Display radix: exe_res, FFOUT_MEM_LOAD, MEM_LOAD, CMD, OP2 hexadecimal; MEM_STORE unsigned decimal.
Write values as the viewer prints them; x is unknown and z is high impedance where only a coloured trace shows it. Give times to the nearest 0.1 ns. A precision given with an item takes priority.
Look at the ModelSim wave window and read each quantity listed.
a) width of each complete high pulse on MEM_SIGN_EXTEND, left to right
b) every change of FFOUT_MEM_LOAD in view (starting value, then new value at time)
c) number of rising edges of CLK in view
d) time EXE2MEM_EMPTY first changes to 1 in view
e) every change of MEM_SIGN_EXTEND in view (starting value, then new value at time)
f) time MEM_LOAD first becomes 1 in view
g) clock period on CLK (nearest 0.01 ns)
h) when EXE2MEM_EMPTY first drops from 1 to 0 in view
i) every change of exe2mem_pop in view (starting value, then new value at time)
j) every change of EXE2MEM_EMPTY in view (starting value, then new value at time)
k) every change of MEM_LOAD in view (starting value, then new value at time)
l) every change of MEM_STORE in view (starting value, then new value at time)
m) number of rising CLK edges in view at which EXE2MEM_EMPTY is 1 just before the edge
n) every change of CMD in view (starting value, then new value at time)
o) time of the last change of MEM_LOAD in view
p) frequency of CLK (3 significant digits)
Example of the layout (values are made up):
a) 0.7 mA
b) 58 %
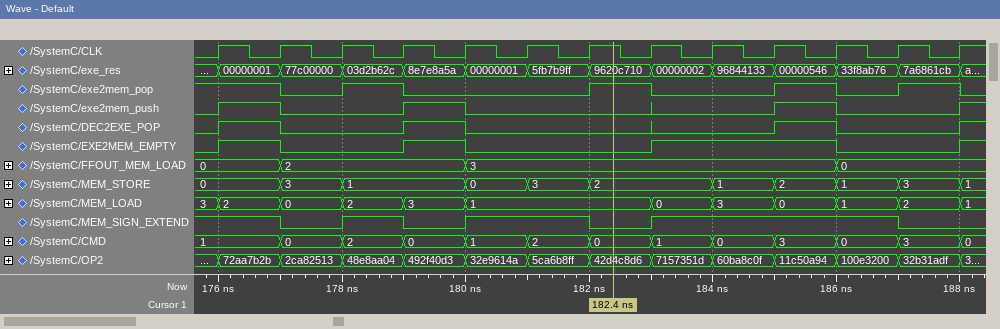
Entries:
a) 1 ns, 2 ns, 4 ns
b) 0, 2 at 177 ns, 3 at 180 ns, 0 at 186 ns
c) 13
d) 176 ns
e) 1, 0 at 177 ns, 1 at 178 ns, 0 at 179 ns, 1 at 180 ns, 0 at 182 ns, 1 at 183 ns, 0 at 187 ns
f) 180 ns
g) 1 ns
h) 177 ns
i) 1, 0 at 177 ns, 1 at 178 ns, 0 at 179 ns, 1 at 182 ns, 0 at 183 ns, 1 at 185 ns, 0 at 186 ns, 1 at 187 ns, 0 at 188 ns
j) 0, 1 at 176 ns, 0 at 177 ns, 1 at 179 ns, 0 at 180 ns, 1 at 183 ns, 0 at 186 ns, 1 at 188 ns
k) 3, 2 at 176 ns, 0 at 177 ns, 2 at 178 ns, 3 at 179 ns, 1 at 180 ns, 0 at 183 ns, 3 at 184 ns, 0 at 185 ns, 1 at 186 ns, 2 at 187 ns, 1 at 188 ns
l) 0, 3 at 177 ns, 1 at 178 ns, 0 at 180 ns, 3 at 181 ns, 2 at 182 ns, 1 at 184 ns, 2 at 185 ns, 1 at 186 ns, 3 at 187 ns, 1 at 188 ns
m) 5
n) 1, 0 at 177 ns, 2 at 178 ns, 0 at 179 ns, 1 at 180 ns, 2 at 181 ns, 0 at 182 ns, 1 at 183 ns, 0 at 184 ns, 3 at 185 ns, 0 at 186 ns, 3 at 187 ns, 0 at 188 ns
o) 188 ns
p) 1.00 GHz
